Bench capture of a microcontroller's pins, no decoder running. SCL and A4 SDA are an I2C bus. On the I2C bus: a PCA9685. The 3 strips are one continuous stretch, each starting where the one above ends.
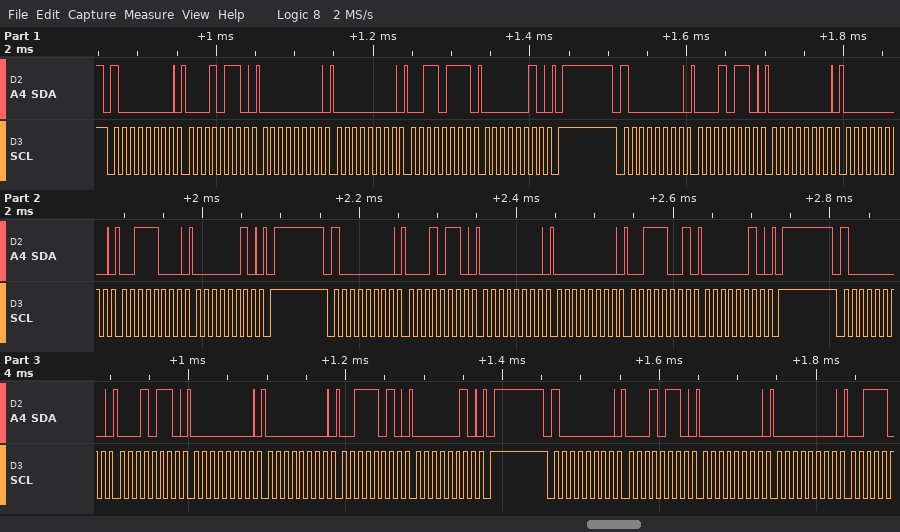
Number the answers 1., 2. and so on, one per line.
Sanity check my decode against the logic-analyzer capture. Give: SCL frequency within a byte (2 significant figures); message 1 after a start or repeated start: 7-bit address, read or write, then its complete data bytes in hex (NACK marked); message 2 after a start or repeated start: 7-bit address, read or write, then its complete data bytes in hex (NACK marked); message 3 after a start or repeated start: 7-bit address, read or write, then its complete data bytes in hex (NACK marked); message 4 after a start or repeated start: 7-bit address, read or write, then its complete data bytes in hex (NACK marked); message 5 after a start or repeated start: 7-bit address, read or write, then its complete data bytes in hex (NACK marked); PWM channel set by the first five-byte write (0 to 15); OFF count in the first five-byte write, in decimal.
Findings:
1. 100 kHz
2. 0x40 write: 16 00 00 37 02
3. 0x40 write: 16 00 00 38 02
4. 0x40 write: 16 00 00 39 02
5. 0x40 write: 16 00 00 3A 02
6. 0x40 write: 16 00 00
7. 4
8. 567
